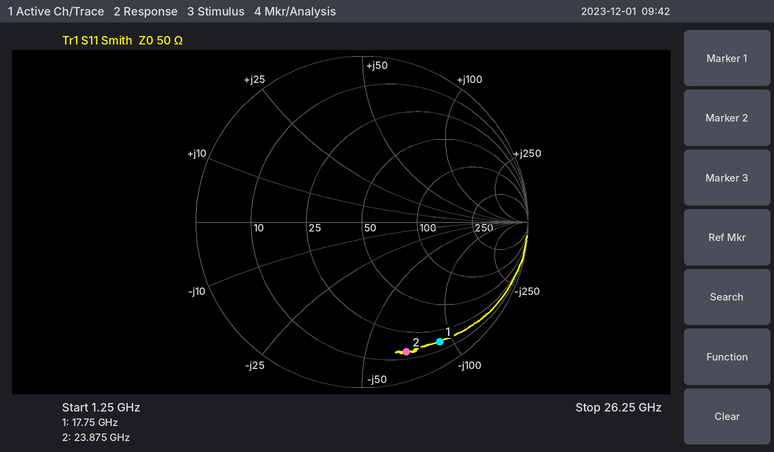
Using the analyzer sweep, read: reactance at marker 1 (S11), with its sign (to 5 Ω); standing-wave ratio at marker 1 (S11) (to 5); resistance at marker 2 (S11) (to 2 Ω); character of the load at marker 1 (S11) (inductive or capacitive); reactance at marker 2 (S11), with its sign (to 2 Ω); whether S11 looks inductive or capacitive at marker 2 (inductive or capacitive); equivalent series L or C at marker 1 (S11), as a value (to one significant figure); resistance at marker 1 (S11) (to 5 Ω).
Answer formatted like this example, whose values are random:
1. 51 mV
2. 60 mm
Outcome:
1. -90 Ω
2. 15
3. 14 Ω
4. capacitive
5. -68 Ω
6. capacitive
7. 100 fF
8. 15 Ω
